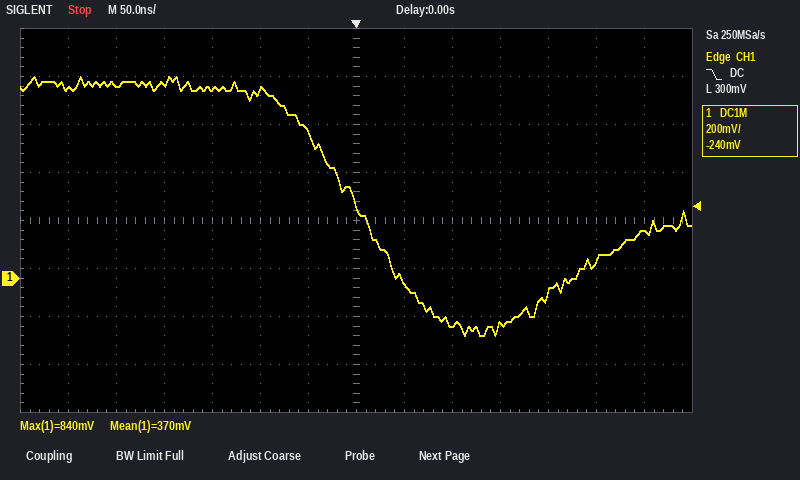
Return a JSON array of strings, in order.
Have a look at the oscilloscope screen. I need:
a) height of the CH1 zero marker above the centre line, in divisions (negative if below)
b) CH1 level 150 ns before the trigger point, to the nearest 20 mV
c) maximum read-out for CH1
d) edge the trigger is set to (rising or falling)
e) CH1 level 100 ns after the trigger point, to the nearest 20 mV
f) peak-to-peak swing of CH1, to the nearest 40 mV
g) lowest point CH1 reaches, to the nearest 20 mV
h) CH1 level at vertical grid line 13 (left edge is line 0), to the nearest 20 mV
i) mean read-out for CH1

["-1.2 div", "780 mV", "840 mV", "falling", "-200 mV", "1.08 V", "-240 mV", "200 mV", "370 mV"]
